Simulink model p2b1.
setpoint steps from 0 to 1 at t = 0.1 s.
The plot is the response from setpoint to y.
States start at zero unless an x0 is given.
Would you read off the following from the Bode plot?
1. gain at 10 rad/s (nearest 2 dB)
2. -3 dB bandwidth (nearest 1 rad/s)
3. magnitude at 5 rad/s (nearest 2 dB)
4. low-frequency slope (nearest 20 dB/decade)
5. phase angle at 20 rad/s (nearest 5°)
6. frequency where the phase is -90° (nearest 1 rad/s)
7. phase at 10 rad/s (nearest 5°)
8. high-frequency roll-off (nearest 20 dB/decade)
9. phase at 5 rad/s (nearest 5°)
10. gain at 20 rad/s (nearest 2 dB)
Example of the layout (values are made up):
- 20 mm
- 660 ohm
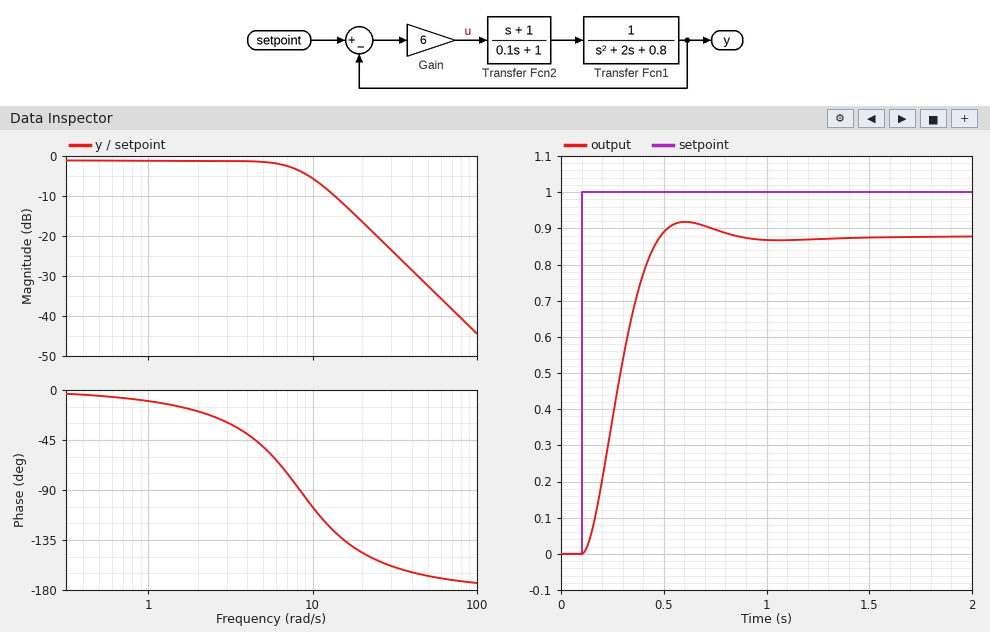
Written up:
- -6 dB
- 9 rad/s
- -2 dB
- 0 dB/decade
- -145°
- 8 rad/s
- -105°
- -40 dB/decade
- -50°
- -16 dB
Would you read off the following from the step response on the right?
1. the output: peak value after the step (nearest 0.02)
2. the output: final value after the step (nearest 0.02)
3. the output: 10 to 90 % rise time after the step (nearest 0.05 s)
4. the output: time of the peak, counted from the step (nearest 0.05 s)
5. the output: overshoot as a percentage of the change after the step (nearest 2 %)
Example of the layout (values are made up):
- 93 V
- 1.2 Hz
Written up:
- 0.92
- 0.88
- 0.25 s
- 0.50 s
- 4 %
